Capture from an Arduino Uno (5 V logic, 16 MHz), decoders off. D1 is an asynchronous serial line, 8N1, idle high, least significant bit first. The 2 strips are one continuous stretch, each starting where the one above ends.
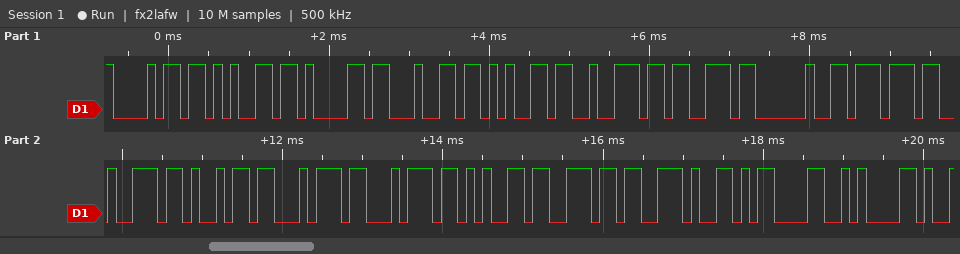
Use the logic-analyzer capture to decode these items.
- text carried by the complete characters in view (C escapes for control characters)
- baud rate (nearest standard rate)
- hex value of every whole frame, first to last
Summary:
"headers written.\r\n"
9600 baud
68 65 61 64 65 72 73 20 77 72 69 74 74 65 6E 2E 0D 0A
